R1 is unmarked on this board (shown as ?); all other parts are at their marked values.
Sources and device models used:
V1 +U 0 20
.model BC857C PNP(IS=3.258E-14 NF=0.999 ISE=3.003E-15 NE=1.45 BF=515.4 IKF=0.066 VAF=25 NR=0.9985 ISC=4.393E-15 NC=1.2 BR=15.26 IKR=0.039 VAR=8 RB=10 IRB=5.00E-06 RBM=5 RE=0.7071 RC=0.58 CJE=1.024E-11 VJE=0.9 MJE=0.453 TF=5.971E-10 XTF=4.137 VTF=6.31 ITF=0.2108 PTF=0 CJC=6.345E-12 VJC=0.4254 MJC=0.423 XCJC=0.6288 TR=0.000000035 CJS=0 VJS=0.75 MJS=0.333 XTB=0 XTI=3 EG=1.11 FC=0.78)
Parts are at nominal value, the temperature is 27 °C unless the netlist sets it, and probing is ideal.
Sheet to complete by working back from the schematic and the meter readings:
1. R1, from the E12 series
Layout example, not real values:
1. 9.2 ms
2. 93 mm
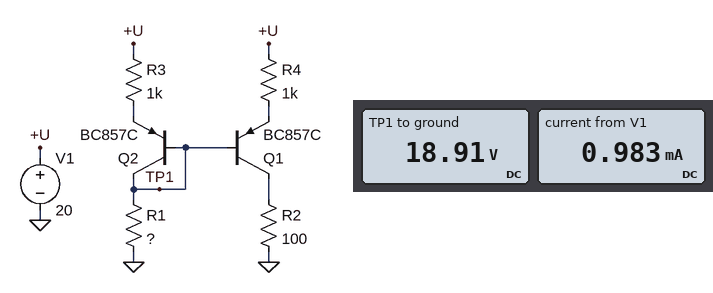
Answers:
1. 39 kΩ
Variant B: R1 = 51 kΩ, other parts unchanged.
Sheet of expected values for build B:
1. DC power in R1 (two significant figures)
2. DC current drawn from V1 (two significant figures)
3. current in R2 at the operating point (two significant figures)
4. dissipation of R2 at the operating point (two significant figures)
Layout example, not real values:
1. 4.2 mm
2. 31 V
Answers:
1. 7.1 mW
2. 760 µA
3. 390 µA
4. 15 µW
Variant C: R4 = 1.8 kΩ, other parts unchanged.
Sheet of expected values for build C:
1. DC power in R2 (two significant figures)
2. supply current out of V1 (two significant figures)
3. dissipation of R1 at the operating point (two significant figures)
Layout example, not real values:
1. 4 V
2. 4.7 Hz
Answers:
1. 8.1 µW
2. 770 µA
3. 9.2 mW
